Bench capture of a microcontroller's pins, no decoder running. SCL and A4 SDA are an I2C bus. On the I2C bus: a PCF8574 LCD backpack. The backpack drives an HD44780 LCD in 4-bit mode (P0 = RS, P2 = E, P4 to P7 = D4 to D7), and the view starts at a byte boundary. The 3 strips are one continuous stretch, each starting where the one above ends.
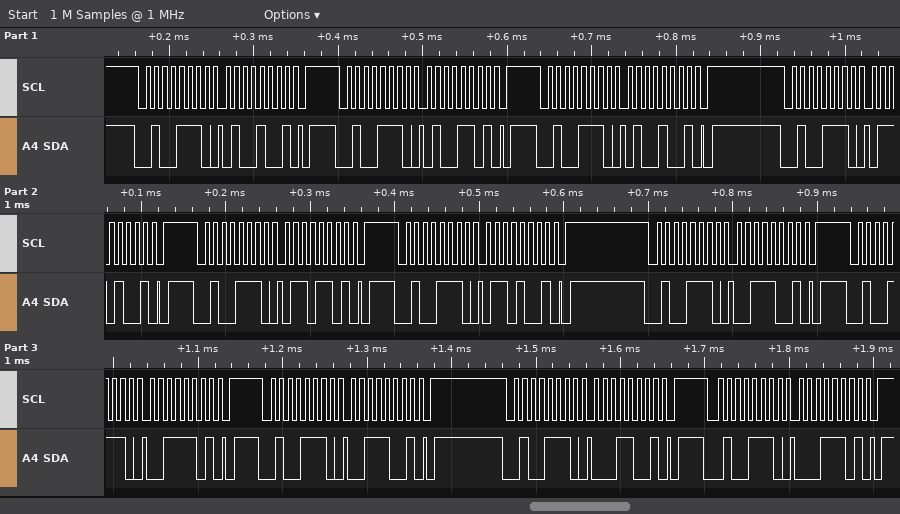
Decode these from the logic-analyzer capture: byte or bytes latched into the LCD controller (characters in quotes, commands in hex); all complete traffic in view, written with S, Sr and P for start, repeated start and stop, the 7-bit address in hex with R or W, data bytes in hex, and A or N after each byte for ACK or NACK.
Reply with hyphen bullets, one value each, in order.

- 'F'
- S 27W A 49 A P S 27W A 4D A P S 27W A 49 A P S 27W A 69 A P S 27W A 6D A P S 27W A 69 A P S 27W A 39 A P S 27W A 3D A P S 27W A 39 A P S 27W A 19 A P S 27W A 1D A P
